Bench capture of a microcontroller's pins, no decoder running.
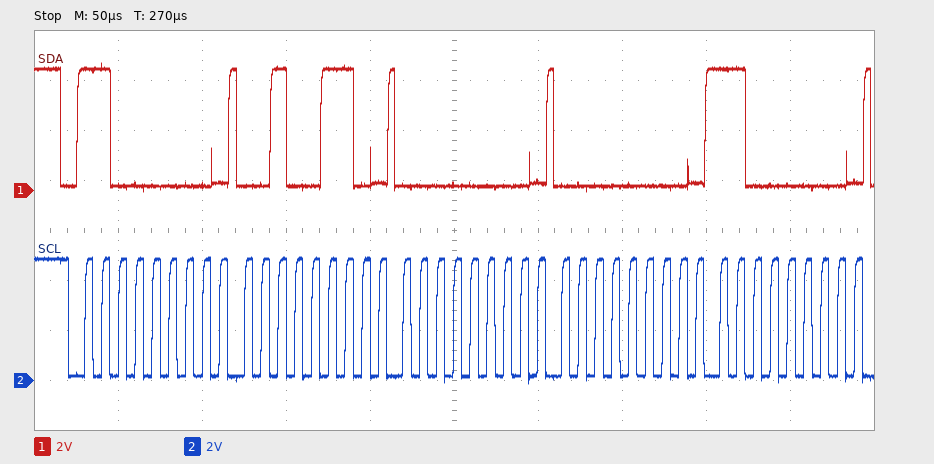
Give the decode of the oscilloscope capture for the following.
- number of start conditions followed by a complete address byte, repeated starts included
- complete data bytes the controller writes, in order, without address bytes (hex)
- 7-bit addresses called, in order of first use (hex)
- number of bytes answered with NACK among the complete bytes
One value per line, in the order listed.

1
26 00 00 C0
0x60
0
